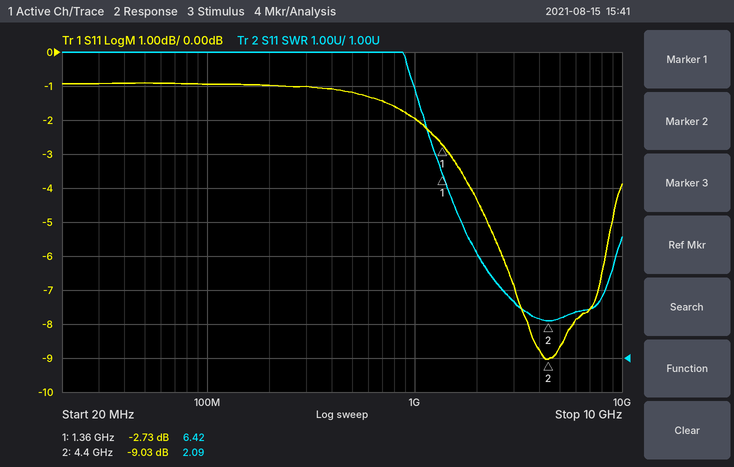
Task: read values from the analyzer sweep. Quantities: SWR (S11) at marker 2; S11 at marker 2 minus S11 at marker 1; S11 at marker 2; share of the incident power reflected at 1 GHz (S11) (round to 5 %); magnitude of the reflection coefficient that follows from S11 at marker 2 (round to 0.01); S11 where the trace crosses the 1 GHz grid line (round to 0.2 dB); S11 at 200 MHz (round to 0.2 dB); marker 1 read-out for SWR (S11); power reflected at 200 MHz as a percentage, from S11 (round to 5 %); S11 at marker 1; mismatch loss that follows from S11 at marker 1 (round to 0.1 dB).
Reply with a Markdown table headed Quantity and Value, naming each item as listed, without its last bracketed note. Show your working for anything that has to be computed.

| Quantity | Value |
|---|---|
| SWR (S11) at marker 2 | 2.09 |
| S11 at marker 2 minus S11 at marker 1 | -9.03 − (-2.73) = -6.30 dB |
| S11 at marker 2 | -9.03 dB |
| share of the incident power reflected at 1 GHz (S11) | 10^(-2/10) ≈ 63.1 %, so 65 % to the nearest 5 % |
| magnitude of the reflection coefficient that follows from S11 at marker 2 | 10^(-9.03/20) ≈ 0.35 |
| S11 where the trace crosses the 1 GHz grid line | -2.0 dB |
| S11 at 200 MHz | -1.0 dB |
| marker 1 read-out for SWR | 6.42 |
| power reflected at 200 MHz as a percentage, from S11 | 10^(-1/10) ≈ 79.4 %, so 80 % to the nearest 5 % |
| S11 at marker 1 | -2.73 dB |
| mismatch loss that follows from S11 at marker 1 | −10 log10(1 − 10^(-2.73/10)) ≈ 3.3 dB |
